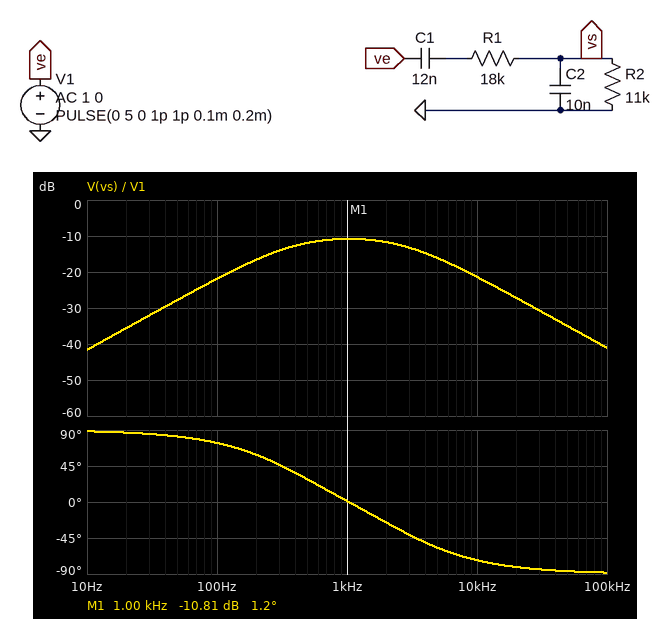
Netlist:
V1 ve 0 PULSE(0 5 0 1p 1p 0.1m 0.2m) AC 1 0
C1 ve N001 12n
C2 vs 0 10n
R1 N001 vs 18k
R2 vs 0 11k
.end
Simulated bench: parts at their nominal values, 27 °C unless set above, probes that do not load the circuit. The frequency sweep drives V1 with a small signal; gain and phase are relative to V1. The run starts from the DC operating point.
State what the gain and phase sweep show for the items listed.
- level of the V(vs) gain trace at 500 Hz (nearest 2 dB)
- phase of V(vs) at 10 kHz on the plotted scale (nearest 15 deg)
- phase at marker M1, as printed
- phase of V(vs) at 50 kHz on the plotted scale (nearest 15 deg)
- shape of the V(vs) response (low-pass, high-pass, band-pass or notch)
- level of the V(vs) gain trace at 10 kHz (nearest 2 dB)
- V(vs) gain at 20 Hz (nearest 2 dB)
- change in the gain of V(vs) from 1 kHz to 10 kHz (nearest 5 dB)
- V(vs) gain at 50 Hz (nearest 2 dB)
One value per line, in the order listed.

-12 dB
-75 deg
1.2 deg
-90 deg
band-pass
-22 dB
-36 dB
-10 dB
-28 dB
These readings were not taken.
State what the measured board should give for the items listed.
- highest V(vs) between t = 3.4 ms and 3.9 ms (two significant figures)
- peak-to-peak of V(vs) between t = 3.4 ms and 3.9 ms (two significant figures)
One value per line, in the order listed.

550 mV
1.1 V
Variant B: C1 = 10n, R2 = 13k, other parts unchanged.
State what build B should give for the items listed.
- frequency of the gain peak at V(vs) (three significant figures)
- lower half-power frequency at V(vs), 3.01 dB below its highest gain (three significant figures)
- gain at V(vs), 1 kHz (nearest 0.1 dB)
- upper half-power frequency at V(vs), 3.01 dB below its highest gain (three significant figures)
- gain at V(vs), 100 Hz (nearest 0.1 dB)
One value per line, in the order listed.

1.04 kHz
326 Hz
-10.6 dB
3.32 kHz
-22.0 dB
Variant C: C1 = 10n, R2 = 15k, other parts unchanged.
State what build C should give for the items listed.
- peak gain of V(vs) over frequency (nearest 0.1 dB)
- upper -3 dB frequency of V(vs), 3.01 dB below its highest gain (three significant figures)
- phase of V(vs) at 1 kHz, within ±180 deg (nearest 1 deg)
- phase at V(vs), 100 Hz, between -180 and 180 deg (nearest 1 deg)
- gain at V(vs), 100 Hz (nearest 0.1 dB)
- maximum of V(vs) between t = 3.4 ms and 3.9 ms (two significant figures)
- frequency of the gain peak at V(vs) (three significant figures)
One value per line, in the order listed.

-10.1 dB
3.13 kHz
-1 deg
73 deg
-20.8 dB
560 mV
969 Hz
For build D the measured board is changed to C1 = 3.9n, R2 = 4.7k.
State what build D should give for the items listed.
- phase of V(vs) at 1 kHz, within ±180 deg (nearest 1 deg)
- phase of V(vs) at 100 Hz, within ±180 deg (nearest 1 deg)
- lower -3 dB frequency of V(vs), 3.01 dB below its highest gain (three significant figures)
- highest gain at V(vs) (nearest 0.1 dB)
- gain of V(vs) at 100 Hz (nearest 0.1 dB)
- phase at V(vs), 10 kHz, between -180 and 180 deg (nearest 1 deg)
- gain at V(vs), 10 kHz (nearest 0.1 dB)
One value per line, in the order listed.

46 deg
85 deg
1.02 kHz
-17.4 dB
-38.8 dB
-55 deg
-22.1 dB
